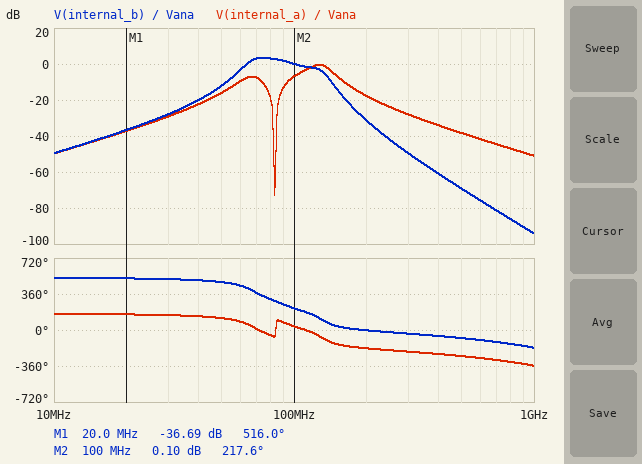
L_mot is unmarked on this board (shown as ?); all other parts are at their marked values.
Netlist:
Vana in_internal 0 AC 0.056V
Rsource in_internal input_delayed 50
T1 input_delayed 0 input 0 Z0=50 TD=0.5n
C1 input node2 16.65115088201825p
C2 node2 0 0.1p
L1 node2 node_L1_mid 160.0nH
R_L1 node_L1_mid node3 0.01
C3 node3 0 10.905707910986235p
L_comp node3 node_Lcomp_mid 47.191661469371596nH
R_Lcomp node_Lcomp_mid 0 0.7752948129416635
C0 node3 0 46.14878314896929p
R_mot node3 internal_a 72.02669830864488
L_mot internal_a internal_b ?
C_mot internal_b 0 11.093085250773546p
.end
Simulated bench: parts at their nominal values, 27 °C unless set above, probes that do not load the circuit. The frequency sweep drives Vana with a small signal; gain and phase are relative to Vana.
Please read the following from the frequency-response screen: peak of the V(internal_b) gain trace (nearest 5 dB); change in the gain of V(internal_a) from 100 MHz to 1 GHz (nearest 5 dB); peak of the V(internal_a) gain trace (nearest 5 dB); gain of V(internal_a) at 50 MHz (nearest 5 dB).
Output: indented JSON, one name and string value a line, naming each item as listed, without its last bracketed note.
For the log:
{
  "peak of the V(internal_b) gain trace": "5 dB",
  "change in the gain of V(internal_a) from 100 MHz to 1 GHz": "-45 dB",
  "peak of the V(internal_a) gain trace": "0 dB",
  "gain of V(internal_a) at 50 MHz": "-15 dB"
}
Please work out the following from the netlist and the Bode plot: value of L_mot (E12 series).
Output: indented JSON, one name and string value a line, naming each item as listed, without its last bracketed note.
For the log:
{
  "value of L_mot": "330 nH"
}
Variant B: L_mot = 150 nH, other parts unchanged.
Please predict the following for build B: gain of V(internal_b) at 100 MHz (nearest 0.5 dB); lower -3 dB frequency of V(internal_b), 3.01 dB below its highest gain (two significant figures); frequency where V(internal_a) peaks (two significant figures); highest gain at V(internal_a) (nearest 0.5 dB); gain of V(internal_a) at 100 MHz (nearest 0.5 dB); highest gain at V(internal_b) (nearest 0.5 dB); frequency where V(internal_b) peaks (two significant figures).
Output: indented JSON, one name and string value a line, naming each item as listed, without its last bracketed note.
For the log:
{
  "gain of V(internal_b) at 100 MHz": "0.5 dB",
  "lower -3 dB frequency of V(internal_b), 3.01 dB below its highest gain": "67 MHz",
  "frequency where V(internal_a) peaks": "73 MHz",
  "highest gain at V(internal_a)": "-2.0 dB",
  "gain of V(internal_a) at 100 MHz": "-9.0 dB",
  "highest gain at V(internal_b)": "2.0 dB",
  "frequency where V(internal_b) peaks": "75 MHz"
}
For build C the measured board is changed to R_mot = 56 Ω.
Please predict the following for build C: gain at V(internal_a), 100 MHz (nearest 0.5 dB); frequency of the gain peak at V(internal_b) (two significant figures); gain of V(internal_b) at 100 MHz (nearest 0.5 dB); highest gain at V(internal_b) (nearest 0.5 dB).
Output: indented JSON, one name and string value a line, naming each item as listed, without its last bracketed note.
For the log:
{
  "gain at V(internal_a), 100 MHz": "-6.0 dB",
  "frequency of the gain peak at V(internal_b)": "72 MHz",
  "gain of V(internal_b) at 100 MHz": "1.0 dB",
  "highest gain at V(internal_b)": "4.5 dB"
}
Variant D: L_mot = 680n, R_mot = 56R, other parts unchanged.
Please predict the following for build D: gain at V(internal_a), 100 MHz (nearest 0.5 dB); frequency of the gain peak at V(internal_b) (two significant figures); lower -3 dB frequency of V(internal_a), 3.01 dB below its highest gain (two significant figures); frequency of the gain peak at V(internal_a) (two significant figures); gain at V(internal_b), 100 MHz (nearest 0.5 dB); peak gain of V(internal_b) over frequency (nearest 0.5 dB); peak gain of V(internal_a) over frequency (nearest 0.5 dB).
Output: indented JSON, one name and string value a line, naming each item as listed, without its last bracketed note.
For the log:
{
  "gain at V(internal_a), 100 MHz": "-1.0 dB",
  "frequency of the gain peak at V(internal_b)": "57 MHz",
  "lower -3 dB frequency of V(internal_a), 3.01 dB below its highest gain": "80 MHz",
  "frequency of the gain peak at V(internal_a)": "120 MHz",
  "gain at V(internal_b), 100 MHz": "-7.0 dB",
  "peak gain of V(internal_b) over frequency": "0 dB",
  "peak gain of V(internal_a) over frequency": "1.5 dB"
}
